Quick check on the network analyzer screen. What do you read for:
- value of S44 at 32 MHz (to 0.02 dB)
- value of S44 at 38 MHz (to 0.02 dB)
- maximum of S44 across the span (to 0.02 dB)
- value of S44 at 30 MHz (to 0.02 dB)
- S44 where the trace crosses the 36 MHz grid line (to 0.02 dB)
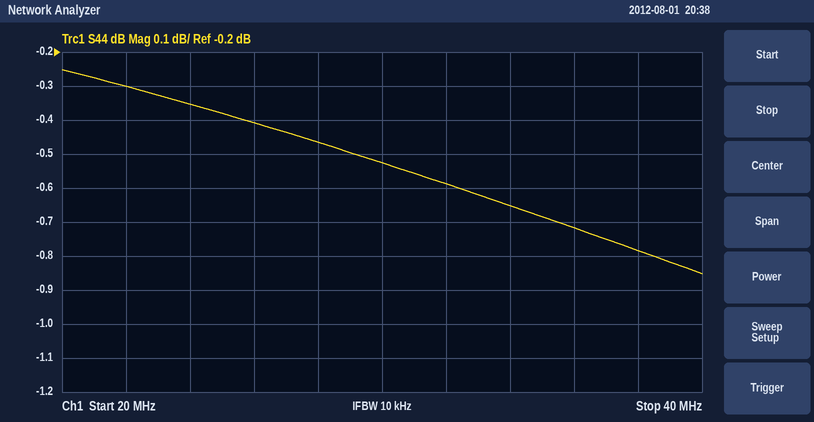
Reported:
-0.58 dB
-0.78 dB
-0.26 dB
-0.52 dB
-0.72 dB
